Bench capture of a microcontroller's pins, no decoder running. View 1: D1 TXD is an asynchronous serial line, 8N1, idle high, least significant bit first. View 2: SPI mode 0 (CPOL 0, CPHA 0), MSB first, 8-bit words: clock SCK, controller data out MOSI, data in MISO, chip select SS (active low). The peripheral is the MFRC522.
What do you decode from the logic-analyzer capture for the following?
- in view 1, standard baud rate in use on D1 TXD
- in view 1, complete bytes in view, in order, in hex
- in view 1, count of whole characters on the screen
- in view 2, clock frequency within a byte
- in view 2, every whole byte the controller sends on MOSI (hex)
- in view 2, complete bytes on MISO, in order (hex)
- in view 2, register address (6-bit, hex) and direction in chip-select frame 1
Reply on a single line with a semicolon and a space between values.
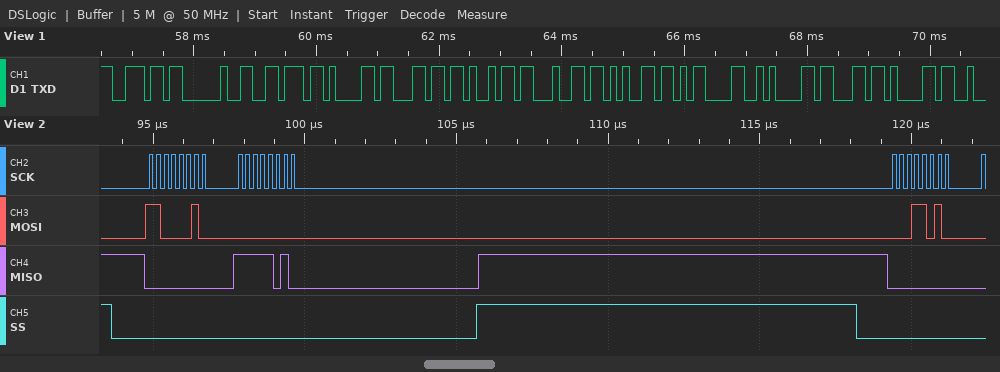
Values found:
9600 baud; 6E 20 76 61 6C 69 64 65 0D 0A 63 61; 12; 4 MHz; C2 00 1A; 00 FA 00; 0x21 read
